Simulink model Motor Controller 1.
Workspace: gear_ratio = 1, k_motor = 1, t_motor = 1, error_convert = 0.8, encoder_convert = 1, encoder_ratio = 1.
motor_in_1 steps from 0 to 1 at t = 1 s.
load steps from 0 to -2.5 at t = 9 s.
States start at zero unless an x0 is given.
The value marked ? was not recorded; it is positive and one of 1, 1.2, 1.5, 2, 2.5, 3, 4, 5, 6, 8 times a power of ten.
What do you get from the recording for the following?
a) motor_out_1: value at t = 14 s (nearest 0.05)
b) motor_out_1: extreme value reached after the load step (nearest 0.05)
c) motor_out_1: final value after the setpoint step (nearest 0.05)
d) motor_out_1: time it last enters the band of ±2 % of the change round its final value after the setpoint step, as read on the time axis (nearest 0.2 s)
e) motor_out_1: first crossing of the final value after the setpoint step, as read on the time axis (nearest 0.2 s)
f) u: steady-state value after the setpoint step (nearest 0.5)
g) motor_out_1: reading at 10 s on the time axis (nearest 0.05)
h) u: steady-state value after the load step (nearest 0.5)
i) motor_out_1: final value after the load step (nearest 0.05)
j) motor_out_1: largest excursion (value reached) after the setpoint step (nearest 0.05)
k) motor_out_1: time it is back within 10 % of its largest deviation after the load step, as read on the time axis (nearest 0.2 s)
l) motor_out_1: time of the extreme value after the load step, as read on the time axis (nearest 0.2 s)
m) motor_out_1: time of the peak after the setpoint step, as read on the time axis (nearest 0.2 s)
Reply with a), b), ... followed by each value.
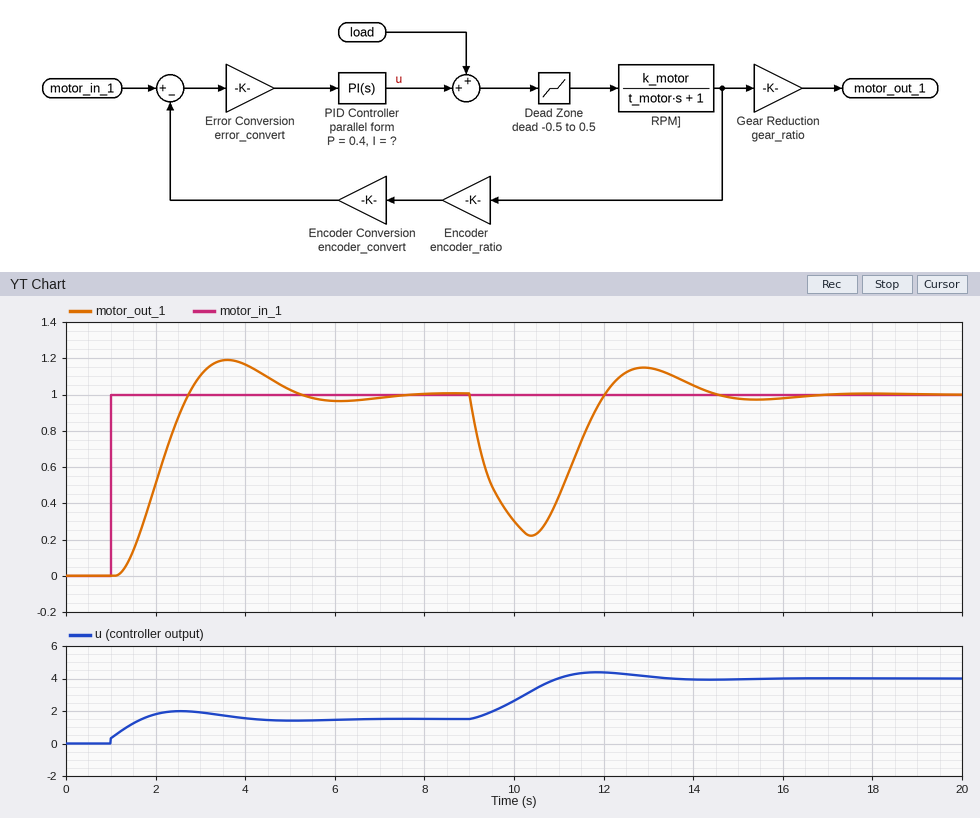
a) 1.05
b) 0.20
c) 1.00
d) 7.0 s
e) 2.8 s
f) 1.5
g) 0.30
h) 4.0
i) 1.00
j) 1.20
k) 13.8 s
l) 10.4 s
m) 3.6 s
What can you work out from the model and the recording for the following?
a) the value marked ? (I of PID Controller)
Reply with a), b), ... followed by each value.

a) 2.5
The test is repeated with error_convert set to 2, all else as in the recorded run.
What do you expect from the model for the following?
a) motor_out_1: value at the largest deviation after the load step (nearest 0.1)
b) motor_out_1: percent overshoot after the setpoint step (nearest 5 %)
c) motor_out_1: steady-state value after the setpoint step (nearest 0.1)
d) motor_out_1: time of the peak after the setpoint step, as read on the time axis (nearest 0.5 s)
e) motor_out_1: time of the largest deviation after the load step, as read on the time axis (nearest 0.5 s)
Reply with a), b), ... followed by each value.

a) 0.4
b) 25 %
c) 1.0
d) 2.5 s
e) 10.0 s
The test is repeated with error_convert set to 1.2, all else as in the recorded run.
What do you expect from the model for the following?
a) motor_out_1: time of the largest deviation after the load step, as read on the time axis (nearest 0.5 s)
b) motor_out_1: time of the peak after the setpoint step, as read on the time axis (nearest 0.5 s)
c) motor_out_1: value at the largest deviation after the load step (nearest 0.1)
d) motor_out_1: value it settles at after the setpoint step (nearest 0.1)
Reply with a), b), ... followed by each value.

a) 10.0 s
b) 3.0 s
c) 0.3
d) 1.0
